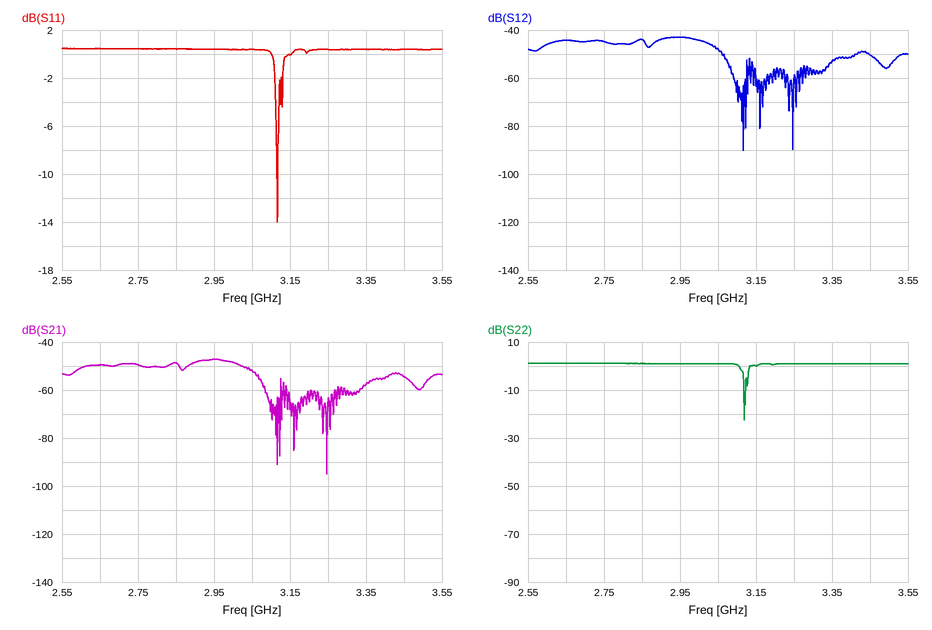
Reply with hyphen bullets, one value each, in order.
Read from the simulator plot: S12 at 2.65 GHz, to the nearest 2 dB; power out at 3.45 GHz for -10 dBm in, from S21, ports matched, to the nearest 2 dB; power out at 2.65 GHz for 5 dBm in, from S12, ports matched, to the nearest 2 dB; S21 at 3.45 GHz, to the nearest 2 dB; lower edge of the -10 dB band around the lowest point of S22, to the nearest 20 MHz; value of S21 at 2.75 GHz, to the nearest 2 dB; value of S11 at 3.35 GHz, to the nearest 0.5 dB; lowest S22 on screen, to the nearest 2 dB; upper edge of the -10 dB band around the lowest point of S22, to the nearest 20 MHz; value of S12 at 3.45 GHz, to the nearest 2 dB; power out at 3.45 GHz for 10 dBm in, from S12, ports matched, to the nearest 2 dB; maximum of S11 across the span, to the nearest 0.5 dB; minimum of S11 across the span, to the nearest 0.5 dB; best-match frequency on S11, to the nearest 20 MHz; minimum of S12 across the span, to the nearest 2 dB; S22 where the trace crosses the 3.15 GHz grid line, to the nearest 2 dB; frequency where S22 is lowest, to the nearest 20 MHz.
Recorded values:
- -44 dB
- -64 dBm
- -40 dBm
- -54 dB
- 3.12 GHz
- -50 dB
- 0.5 dB
- -22 dB
- 3.12 GHz
- -50 dB
- -40 dBm
- 0.5 dB
- -14.0 dB
- 3.12 GHz
- -90 dB
- 0 dB
- 3.12 GHz
